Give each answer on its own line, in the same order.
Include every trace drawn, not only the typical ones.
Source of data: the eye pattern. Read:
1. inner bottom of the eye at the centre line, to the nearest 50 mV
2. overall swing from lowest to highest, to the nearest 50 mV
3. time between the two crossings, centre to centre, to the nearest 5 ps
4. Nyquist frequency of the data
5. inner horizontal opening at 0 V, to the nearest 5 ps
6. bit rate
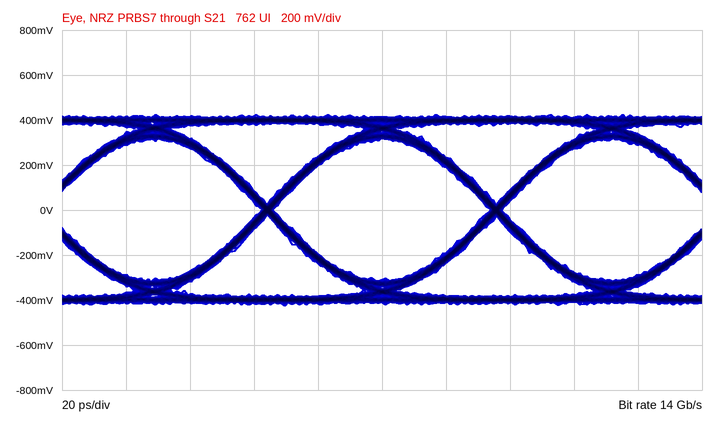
-300 mV
850 mV
70 ps
7 GHz
70 ps
14 Gb/s
